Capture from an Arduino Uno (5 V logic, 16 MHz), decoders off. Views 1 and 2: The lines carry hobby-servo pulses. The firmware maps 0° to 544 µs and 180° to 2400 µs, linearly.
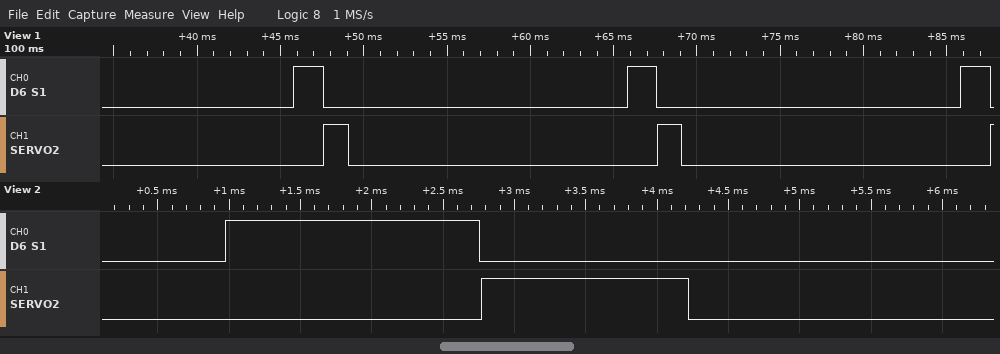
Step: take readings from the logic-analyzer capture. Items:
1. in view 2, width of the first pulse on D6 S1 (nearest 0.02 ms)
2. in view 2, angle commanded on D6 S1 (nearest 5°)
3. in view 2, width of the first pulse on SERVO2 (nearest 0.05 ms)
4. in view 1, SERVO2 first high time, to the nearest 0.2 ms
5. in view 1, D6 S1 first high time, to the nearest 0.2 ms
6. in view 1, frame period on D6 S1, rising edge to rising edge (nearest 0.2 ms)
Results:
1.78 ms
120°
1.45 ms
1.4 ms
1.8 ms
20.0 ms
